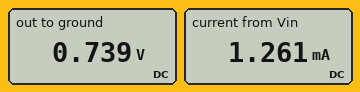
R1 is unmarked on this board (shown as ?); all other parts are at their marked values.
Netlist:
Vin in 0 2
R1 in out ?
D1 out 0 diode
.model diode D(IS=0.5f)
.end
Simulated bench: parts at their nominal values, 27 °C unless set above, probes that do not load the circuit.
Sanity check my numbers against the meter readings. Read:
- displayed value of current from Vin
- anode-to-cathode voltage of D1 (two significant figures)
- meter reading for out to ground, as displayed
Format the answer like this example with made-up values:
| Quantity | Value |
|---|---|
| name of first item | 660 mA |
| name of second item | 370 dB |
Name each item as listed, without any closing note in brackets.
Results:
| Quantity | Value |
|---|---|
| displayed value of current from Vin | 1.261 mA |
| anode-to-cathode voltage of D1 | 740 mV |
| meter reading for out to ground, as displayed | 0.739 V |
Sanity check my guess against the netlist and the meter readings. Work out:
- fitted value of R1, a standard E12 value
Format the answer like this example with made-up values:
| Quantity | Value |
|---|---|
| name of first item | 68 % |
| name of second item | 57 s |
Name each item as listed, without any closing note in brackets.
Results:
| Quantity | Value |
|---|---|
| fitted value of R1, a standard E12 value | 1 kΩ |
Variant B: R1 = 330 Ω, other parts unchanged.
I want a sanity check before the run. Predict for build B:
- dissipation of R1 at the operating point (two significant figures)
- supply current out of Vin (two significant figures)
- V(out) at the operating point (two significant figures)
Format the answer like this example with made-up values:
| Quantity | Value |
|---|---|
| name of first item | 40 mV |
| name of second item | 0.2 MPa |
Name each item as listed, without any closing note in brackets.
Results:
| Quantity | Value |
|---|---|
| dissipation of R1 at the operating point | 4.6 mW |
| supply current out of Vin | 3.7 mA |
| V(out) at the operating point | 770 mV |
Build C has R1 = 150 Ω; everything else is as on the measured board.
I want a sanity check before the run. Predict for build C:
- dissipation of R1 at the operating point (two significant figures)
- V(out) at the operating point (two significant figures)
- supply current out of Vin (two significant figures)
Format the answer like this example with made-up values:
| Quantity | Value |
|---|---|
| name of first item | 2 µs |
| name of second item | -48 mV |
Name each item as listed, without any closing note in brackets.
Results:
| Quantity | Value |
|---|---|
| dissipation of R1 at the operating point | 9.8 mW |
| V(out) at the operating point | 790 mV |
| supply current out of Vin | 8.1 mA |
